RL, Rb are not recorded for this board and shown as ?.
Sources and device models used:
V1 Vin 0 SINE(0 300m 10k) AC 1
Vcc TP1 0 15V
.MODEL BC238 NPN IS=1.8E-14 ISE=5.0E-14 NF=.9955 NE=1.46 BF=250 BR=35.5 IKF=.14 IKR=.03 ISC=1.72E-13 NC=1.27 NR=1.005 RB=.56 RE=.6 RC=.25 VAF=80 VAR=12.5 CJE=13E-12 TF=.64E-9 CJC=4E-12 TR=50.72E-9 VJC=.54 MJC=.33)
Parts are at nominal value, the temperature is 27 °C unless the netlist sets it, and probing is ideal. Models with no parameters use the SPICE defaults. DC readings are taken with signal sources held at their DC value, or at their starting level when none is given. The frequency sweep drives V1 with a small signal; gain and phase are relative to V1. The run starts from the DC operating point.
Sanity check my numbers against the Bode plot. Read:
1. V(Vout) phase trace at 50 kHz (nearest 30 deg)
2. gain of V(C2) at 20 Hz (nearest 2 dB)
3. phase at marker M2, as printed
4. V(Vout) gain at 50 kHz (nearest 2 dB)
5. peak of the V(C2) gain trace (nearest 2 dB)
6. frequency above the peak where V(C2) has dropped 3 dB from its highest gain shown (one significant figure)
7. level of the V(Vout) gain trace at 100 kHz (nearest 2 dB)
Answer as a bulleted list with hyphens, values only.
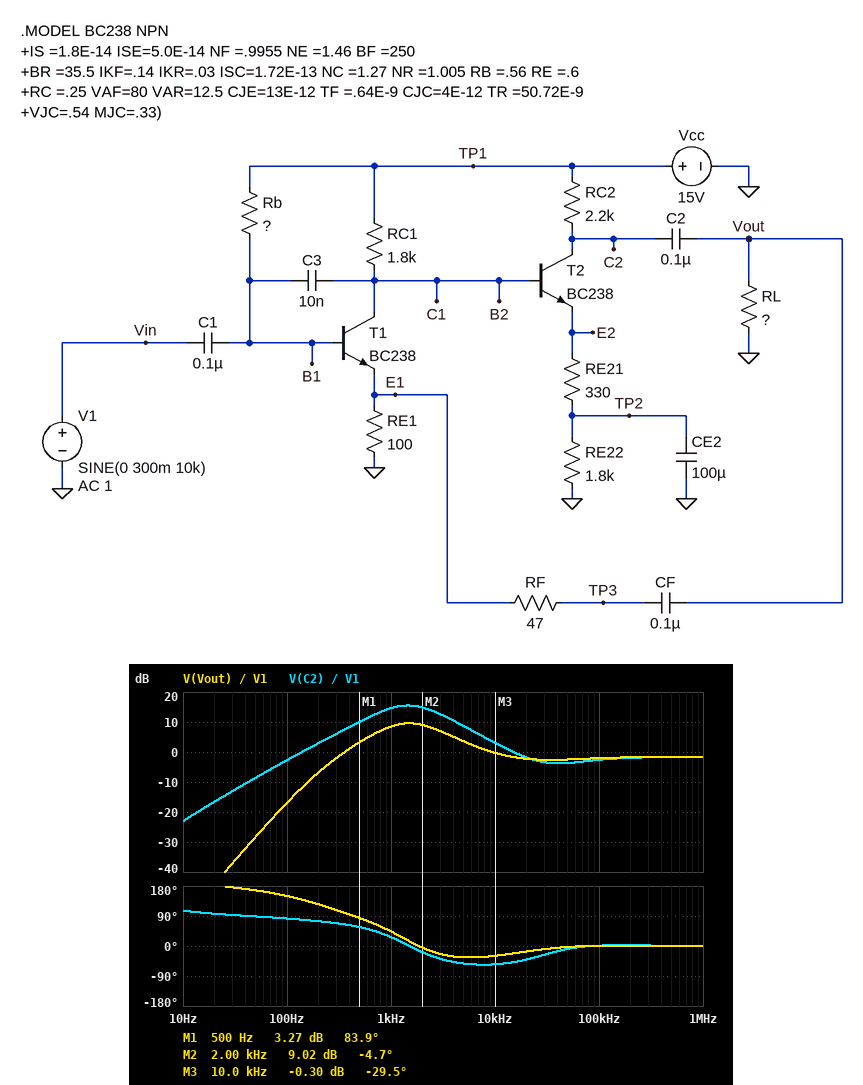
- 0 deg
- -16 dB
- -4.7 deg
- -2 dB
- 16 dB
- 3 kHz
- -2 dB
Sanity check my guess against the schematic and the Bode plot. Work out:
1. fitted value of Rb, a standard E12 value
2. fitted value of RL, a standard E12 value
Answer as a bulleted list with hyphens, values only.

- 270 kΩ
- 3.3 kΩ
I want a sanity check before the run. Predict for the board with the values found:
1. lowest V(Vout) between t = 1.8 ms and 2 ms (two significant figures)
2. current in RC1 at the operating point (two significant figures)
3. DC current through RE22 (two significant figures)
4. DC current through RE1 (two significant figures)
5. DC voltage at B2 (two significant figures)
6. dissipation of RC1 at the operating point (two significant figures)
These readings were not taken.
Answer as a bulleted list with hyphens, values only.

- -380 mV
- 7.8 mA
- 150 µA
- 7.9 mA
- 910 mV
- 110 mW
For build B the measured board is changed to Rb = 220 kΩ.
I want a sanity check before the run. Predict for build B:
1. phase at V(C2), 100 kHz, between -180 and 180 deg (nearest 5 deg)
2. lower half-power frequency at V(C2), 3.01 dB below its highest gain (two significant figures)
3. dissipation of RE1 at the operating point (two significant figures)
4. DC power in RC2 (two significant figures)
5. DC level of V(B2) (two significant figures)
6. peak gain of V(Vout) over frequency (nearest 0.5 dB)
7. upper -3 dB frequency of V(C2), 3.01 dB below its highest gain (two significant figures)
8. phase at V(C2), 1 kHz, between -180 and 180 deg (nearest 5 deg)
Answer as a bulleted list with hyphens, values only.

- 5 deg
- 850 Hz
- 6.2 mW
- 45 µW
- 890 mV
- 3.5 dB
- 4.9 kHz
- 40 deg
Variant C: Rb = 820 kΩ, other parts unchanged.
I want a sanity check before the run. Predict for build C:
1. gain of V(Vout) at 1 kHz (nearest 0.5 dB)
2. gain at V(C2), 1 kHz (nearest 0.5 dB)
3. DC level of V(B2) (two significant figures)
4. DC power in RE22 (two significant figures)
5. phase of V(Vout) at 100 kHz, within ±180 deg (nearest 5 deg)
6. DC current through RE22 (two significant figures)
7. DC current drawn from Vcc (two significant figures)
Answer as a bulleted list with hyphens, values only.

- -29.0 dB
- -3.5 dB
- 8.2 V
- 22 mW
- 20 deg
- 3.5 mA
- 7.2 mA
